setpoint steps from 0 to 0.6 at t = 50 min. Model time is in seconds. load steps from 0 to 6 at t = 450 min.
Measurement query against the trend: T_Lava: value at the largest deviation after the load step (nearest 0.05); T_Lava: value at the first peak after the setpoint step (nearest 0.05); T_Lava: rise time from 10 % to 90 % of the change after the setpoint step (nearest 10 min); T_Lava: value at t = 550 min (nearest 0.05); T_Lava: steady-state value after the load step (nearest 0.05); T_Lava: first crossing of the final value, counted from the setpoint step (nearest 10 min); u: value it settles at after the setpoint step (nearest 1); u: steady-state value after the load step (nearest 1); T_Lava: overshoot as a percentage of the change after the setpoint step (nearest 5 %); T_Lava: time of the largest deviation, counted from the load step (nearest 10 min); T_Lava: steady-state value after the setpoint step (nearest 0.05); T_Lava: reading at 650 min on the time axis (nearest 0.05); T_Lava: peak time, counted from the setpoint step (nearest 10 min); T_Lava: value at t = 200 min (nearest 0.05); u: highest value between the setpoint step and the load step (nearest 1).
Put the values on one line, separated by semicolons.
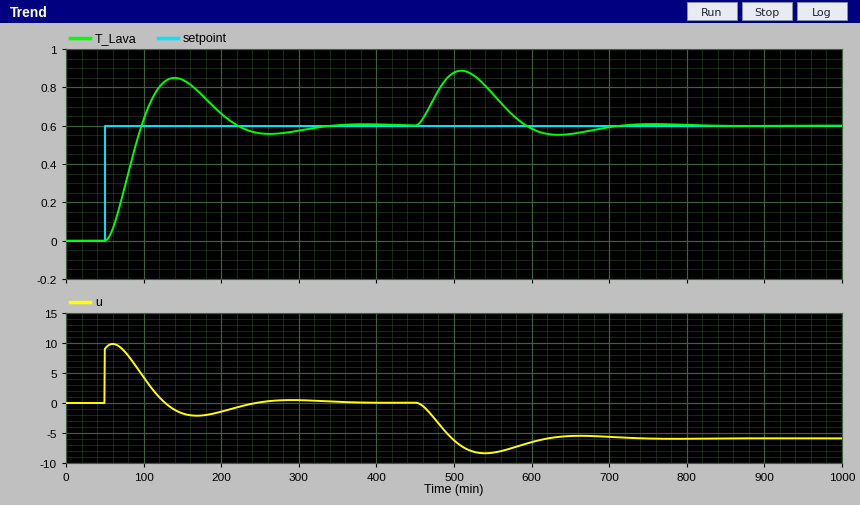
0.90; 0.85; 30 min; 0.75; 0.60; 50 min; 0; -6; 40 %; 60 min; 0.60; 0.55; 90 min; 0.65; 10
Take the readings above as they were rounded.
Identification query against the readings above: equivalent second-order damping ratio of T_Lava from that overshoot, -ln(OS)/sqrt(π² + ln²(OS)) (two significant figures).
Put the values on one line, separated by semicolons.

0.28
